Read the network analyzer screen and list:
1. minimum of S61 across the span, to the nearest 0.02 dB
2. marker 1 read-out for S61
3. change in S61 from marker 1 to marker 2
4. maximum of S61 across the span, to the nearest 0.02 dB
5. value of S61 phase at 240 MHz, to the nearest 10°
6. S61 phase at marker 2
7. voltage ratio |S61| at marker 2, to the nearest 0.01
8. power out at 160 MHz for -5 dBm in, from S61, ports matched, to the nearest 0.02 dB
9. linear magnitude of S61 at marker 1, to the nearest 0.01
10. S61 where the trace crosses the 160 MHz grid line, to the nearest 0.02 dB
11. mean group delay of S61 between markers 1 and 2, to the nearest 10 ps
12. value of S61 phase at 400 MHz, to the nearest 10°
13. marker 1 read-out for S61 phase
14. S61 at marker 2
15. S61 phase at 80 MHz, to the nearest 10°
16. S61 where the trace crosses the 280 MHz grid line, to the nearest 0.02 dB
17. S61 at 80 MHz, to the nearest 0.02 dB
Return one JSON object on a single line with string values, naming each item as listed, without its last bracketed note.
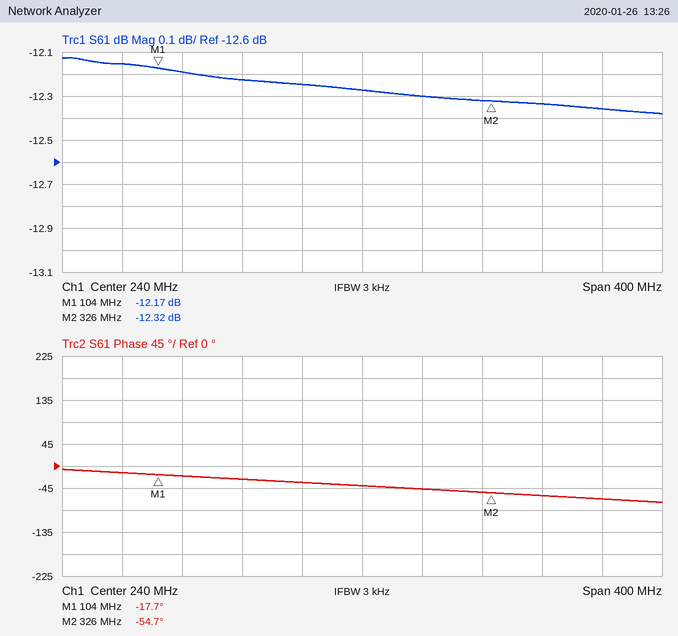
{"minimum of S61 across the span, to the nearest 0.02 dB": "-12.38 dB", "marker 1 read-out for S61": "-12.17 dB", "change in S61 from marker 1 to marker 2": "-0.15 dB", "maximum of S61 across the span, to the nearest 0.02 dB": "-12.12 dB", "value of S61 phase at 240 MHz, to the nearest 10°": "-40°", "S61 phase at marker 2": "-54.7°", "voltage ratio |S61| at marker 2, to the nearest 0.01": "0.24", "power out at 160 MHz for -5 dBm in, from S61, ports matched, to the nearest 0.02 dB": "-17.22 dBm", "linear magnitude of S61 at marker 1, to the nearest 0.01": "0.25", "S61 where the trace crosses the 160 MHz grid line, to the nearest 0.02 dB": "-12.22 dB", "mean group delay of S61 between markers 1 and 2, to the nearest 10 ps": "460 ps", "value of S61 phase at 400 MHz, to the nearest 10°": "-70°", "marker 1 read-out for S61 phase": "-17.7°", "S61 at marker 2": "-12.32 dB", "S61 phase at 80 MHz, to the nearest 10°": "-10°", "S61 where the trace crosses the 280 MHz grid line, to the nearest 0.02 dB": "-12.30 dB", "S61 at 80 MHz, to the nearest 0.02 dB": "-12.16 dB"}
